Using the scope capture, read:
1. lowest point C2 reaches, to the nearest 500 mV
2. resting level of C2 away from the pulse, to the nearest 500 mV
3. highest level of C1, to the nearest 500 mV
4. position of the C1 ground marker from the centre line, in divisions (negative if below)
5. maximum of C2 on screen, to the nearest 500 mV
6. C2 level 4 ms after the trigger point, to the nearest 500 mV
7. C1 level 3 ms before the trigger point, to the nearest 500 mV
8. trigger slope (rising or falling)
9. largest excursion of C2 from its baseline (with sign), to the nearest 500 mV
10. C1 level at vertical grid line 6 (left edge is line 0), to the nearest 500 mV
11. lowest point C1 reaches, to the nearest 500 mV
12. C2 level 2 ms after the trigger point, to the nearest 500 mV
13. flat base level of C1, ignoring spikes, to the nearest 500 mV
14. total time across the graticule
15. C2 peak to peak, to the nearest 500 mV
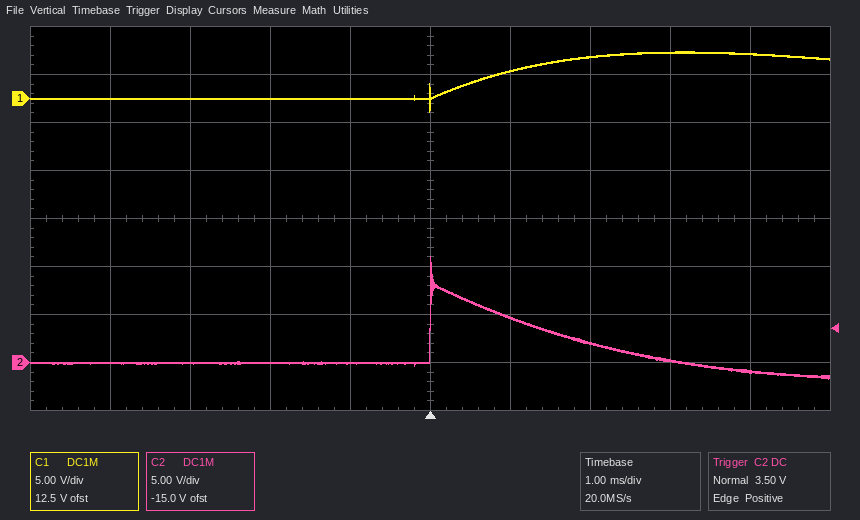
-1.5 V
0.0 V
5.0 V
+2.5 div
11.0 V
-1.0 V
0.0 V
rising
+11.0 V
3.0 V
-1.5 V
2.0 V
0.0 V
10 ms
12.5 V
